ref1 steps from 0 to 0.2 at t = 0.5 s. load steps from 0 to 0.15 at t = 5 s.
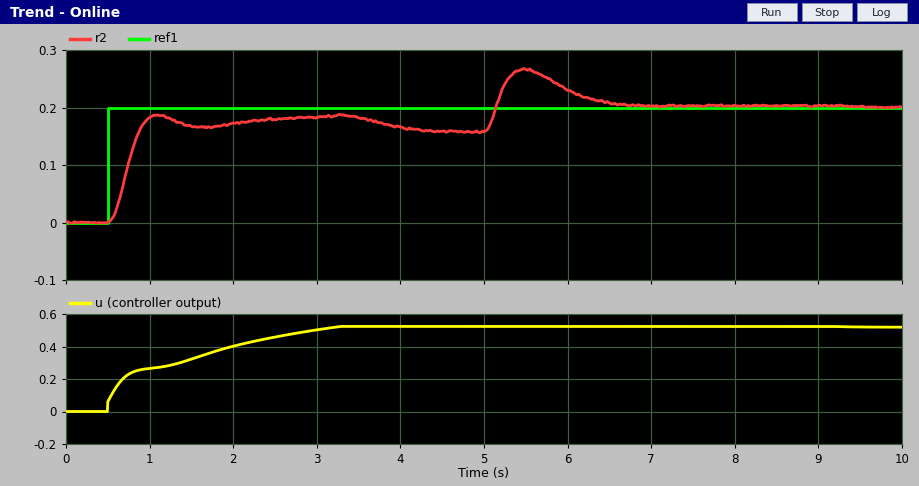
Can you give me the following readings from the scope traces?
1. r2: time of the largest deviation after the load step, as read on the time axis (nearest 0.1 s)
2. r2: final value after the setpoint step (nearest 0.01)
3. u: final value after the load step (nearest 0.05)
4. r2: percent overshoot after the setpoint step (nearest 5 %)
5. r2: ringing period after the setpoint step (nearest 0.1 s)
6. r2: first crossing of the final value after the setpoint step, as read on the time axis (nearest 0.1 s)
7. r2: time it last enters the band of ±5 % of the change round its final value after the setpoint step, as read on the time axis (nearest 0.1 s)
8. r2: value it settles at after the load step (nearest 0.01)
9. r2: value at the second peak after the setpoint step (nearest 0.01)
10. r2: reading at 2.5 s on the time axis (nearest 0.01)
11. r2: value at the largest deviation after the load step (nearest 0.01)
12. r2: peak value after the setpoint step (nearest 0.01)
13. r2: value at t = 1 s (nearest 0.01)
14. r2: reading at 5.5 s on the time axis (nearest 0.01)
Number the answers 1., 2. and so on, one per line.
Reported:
1. 5.5 s
2. 0.16
3. 0.50
4. 20 %
5. 2.2 s
6. 0.9 s
7. 4.0 s
8. 0.20
9. 0.19
10. 0.18
11. 0.27
12. 0.19
13. 0.18
14. 0.27
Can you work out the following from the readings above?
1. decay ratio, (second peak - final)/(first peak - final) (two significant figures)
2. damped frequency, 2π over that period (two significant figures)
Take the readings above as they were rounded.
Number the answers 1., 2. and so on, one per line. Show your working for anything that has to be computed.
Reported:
1. (0.19 - 0.16) / (0.19 - 0.16) = 1.0
2. 2π / 2.2 = 2.9 rad/s
